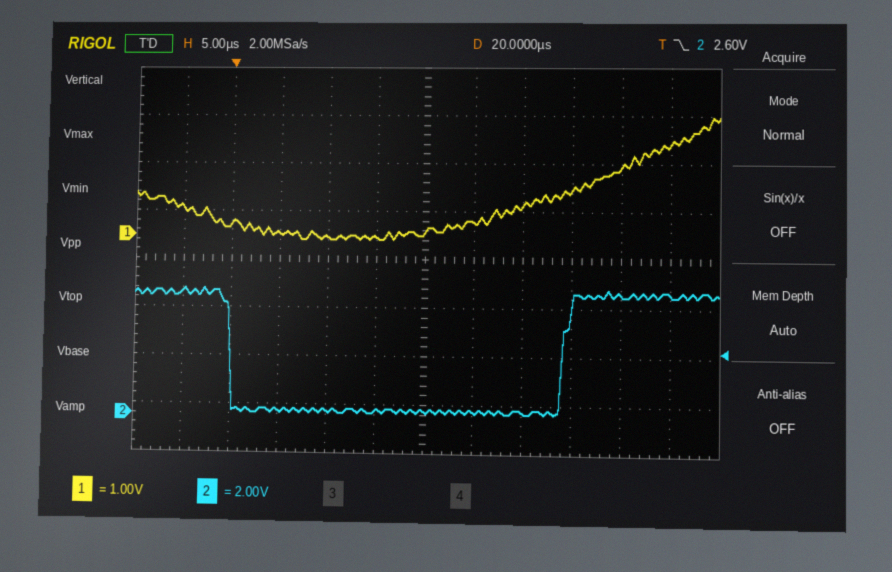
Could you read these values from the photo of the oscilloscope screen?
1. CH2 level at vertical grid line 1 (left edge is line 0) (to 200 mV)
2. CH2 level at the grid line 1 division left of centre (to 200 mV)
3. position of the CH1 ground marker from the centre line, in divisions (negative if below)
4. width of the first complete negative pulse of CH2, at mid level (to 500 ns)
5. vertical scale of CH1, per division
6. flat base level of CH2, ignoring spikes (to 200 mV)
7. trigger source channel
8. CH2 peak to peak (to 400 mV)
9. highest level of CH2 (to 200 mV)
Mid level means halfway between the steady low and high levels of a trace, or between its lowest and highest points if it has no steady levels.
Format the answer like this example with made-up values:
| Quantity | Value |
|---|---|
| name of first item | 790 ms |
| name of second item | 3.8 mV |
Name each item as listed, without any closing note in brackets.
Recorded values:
| Quantity | Value |
|---|---|
| CH2 level at vertical grid line 1 (left edge is line 0) | 5.0 V |
| CH2 level at the grid line 1 division left of centre | 200 mV |
| position of the CH1 ground marker from the centre line, in divisions | +0.5 div |
| width of the first complete negative pulse of CH2, at mid level | 34.0 µs |
| vertical scale of CH1, per division | 1 V |
| flat base level of CH2, ignoring spikes | 200 mV |
| trigger source channel | CH2 |
| CH2 peak to peak | 5.2 V |
| highest level of CH2 | 5.2 V |
